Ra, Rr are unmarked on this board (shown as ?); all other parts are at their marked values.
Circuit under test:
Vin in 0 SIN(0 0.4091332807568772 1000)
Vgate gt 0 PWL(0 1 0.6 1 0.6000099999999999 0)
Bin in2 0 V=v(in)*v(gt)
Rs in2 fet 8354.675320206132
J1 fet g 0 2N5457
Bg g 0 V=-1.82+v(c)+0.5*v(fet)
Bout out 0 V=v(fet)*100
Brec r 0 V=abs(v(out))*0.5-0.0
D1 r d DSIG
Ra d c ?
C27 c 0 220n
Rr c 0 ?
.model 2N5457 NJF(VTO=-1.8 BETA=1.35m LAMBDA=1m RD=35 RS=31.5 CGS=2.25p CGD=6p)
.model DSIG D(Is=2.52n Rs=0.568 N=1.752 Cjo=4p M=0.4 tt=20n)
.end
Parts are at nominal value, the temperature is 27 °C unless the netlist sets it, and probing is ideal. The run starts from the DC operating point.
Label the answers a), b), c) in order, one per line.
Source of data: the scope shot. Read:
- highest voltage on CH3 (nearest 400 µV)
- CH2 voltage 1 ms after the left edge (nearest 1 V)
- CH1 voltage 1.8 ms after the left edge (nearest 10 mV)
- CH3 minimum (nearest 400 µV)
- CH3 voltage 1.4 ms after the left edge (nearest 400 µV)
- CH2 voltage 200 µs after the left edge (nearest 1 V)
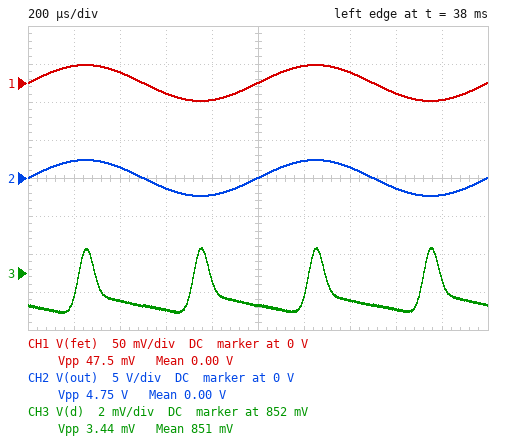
a) 853.2 mV
b) 0 V
c) -20 mV
d) 850.0 mV
e) 850.4 mV
f) 2 V
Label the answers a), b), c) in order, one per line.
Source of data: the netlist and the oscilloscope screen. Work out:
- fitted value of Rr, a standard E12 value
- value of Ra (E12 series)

a) 1.5 MΩ
b) 820 Ω
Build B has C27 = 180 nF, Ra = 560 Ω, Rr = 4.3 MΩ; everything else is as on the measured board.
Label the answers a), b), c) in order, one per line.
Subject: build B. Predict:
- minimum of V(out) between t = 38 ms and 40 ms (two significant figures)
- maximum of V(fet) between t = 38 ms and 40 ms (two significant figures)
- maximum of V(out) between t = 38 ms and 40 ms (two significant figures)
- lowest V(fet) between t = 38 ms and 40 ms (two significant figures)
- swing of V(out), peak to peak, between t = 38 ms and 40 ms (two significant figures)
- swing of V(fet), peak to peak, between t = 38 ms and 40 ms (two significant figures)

a) -2.3 V
b) 23 mV
c) 2.3 V
d) -23 mV
e) 4.6 V
f) 46 mV
